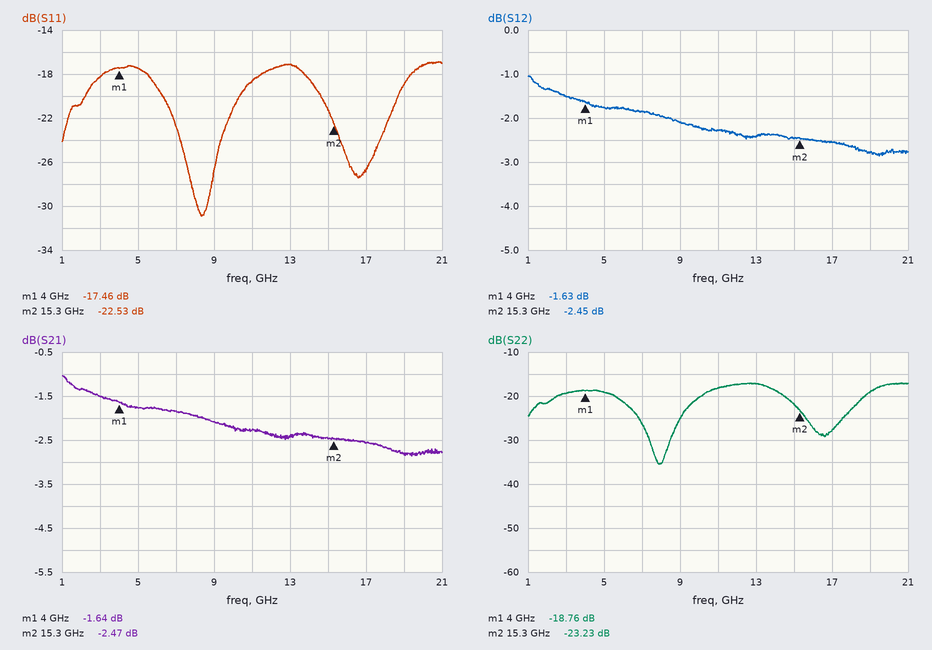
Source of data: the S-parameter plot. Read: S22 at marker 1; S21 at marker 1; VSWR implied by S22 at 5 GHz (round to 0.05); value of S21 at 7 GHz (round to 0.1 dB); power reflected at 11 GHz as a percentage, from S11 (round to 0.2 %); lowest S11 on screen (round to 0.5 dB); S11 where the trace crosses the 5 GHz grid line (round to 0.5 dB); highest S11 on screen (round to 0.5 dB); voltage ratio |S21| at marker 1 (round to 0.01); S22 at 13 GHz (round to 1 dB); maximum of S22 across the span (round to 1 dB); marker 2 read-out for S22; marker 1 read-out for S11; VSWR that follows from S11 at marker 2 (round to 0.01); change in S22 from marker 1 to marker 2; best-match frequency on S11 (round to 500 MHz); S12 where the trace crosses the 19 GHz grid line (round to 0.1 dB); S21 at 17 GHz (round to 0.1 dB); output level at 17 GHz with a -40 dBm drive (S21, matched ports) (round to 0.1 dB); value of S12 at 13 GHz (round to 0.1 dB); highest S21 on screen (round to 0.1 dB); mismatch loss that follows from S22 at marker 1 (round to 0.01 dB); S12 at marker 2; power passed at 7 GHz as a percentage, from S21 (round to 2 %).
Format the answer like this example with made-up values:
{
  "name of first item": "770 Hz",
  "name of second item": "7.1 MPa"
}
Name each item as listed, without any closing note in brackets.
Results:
{
  "S22 at marker 1": "-18.76 dB",
  "S21 at marker 1": "-1.64 dB",
  "VSWR implied by S22 at 5 GHz": "1.25",
  "value of S21 at 7 GHz": "-1.8 dB",
  "power reflected at 11 GHz as a percentage, from S11": "1.4 %",
  "lowest S11 on screen": "-31.0 dB",
  "S11 where the trace crosses the 5 GHz grid line": "-17.5 dB",
  "highest S11 on screen": "-17.0 dB",
  "voltage ratio |S21| at marker 1": "0.83",
  "S22 at 13 GHz": "-17 dB",
  "maximum of S22 across the span": "-17 dB",
  "marker 2 read-out for S22": "-23.23 dB",
  "marker 1 read-out for S11": "-17.46 dB",
  "VSWR that follows from S11 at marker 2": "1.16",
  "change in S22 from marker 1 to marker 2": "-4.47 dB",
  "best-match frequency on S11": "8.5 GHz",
  "S12 where the trace crosses the 19 GHz grid line": "-2.8 dB",
  "S21 at 17 GHz": "-2.6 dB",
  "output level at 17 GHz with a -40 dBm drive (S21, matched ports)": "-42.6 dBm",
  "value of S12 at 13 GHz": "-2.4 dB",
  "highest S21 on screen": "-1.0 dB",
  "mismatch loss that follows from S22 at marker 1": "0.06 dB",
  "S12 at marker 2": "-2.45 dB",
  "power passed at 7 GHz as a percentage, from S21": "66 %"
}
